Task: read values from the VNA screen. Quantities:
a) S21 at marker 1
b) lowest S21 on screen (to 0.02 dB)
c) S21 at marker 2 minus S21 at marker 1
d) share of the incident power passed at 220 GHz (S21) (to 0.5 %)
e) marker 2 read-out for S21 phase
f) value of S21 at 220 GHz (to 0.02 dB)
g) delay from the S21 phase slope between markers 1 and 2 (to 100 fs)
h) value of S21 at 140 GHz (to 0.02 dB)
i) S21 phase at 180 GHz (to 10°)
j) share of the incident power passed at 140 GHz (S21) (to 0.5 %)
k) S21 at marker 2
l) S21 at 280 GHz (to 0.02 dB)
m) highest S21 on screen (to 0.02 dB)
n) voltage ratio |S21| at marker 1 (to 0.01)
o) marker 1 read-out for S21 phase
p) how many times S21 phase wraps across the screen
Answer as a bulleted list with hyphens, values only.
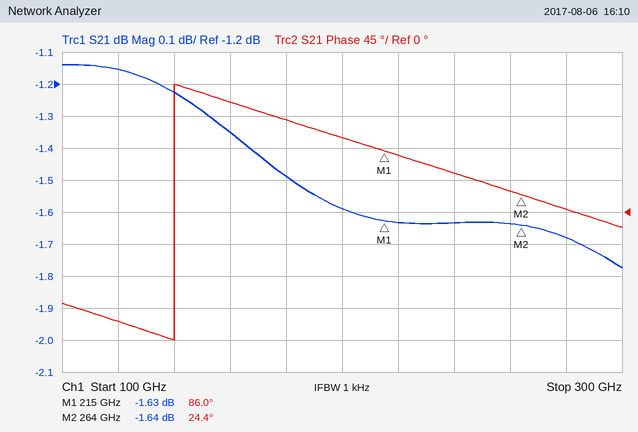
- -1.63 dB
- -1.78 dB
- -0.01 dB
- 68.5 %
- 24.4°
- -1.64 dB
- 3.5 ps
- -1.22 dB
- 130°
- 75.5 %
- -1.64 dB
- -1.68 dB
- -1.14 dB
- 0.83
- 86.0°
- 1
